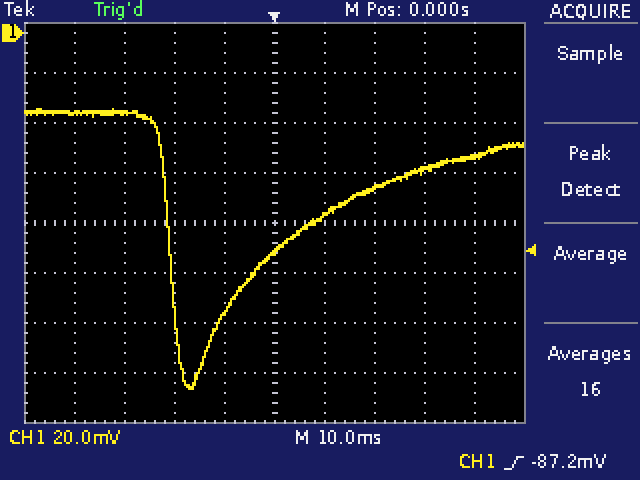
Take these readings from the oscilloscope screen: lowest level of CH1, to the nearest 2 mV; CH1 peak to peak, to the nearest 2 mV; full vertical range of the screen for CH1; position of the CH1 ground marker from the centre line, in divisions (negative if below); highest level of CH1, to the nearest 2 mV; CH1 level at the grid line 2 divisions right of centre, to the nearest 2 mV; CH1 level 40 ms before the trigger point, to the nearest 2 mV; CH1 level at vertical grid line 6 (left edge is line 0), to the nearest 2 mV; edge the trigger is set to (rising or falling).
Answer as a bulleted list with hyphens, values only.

- -142 mV
- 112 mV
- 160 mV
- +3.8 div
- -30 mV
- -62 mV
- -32 mV
- -74 mV
- rising
